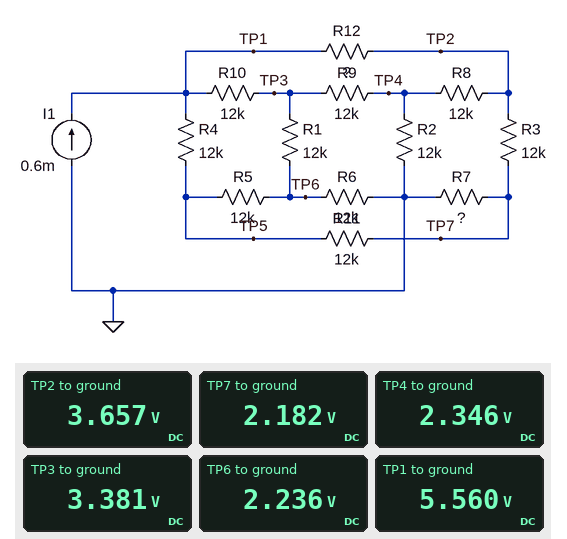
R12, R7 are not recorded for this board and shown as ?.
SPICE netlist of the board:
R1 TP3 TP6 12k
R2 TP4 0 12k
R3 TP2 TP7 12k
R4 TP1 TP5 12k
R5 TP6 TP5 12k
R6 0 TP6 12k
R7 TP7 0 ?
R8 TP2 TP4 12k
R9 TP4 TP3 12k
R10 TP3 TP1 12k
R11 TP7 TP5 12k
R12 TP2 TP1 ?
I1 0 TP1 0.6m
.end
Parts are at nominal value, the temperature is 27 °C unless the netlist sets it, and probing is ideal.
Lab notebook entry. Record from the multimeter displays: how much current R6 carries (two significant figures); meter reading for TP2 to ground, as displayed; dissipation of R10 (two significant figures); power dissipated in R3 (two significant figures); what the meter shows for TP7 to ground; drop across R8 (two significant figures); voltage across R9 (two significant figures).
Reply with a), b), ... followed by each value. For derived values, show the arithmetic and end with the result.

a) (2.236 V) / 12 kΩ = 190 µA
b) 3.657 V
c) (5.56 V - 3.381 V)^2 / 12 kΩ = 400 µW
d) (3.657 V - 2.182 V)^2 / 12 kΩ = 180 µW
e) 2.182 V
f) 3.657 V - 2.346 V = 1.3 V
g) 3.381 V - 2.346 V = 1.0 V
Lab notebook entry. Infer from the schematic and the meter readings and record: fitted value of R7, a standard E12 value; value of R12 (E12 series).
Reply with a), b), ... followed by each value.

a) 10 kΩ
b) 8.2 kΩ
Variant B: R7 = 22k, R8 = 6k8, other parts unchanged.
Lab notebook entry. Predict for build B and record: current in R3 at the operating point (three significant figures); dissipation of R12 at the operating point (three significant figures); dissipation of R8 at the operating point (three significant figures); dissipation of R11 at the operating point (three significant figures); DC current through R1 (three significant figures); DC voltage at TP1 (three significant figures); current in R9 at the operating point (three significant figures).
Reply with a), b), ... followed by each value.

a) 76.4 µA
b) 480 µW
c) 186 µW
d) 51.6 µW
e) 105 µA
f) 6.02 V
g) 77.2 µA
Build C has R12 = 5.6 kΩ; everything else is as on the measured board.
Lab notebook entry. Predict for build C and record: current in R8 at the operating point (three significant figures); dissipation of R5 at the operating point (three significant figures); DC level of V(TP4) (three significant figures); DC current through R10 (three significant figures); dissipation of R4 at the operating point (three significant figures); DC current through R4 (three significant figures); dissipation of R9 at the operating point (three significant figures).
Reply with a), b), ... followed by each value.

a) 123 µA
b) 93.1 µW
c) 2.38 V
d) 168 µA
e) 358 µW
f) 173 µA
g) 68.3 µW
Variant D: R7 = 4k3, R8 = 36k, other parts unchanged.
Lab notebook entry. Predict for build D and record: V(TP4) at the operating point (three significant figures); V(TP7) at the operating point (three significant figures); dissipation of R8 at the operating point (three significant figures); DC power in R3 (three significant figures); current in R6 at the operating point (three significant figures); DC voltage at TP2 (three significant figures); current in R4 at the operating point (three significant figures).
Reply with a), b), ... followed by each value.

a) 1.73 V
b) 1.28 V
c) 73.0 µW
d) 359 µW
e) 158 µA
f) 3.35 V
g) 197 µA
